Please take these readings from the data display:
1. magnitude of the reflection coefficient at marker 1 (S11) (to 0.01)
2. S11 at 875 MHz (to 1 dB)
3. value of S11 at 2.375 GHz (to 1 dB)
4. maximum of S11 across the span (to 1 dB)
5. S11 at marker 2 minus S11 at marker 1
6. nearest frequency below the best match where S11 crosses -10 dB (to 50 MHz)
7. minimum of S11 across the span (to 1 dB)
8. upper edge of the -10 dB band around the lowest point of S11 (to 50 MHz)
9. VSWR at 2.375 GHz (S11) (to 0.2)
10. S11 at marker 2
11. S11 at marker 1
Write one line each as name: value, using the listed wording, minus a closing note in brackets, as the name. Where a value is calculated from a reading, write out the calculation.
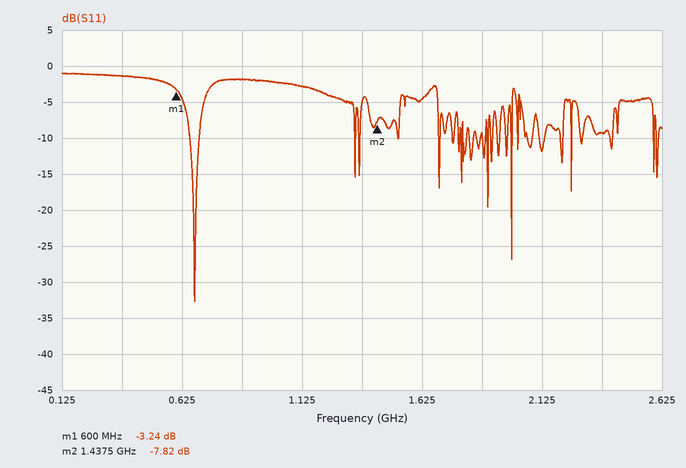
magnitude of the reflection coefficient at marker 1 (S11): 10^(-3.24/20) ≈ 0.69
S11 at 875 MHz: -2 dB
value of S11 at 2.375 GHz: -9 dB
maximum of S11 across the span: -1 dB
S11 at marker 2 minus S11 at marker 1: -7.82 − (-3.24) = -4.58 dB
nearest frequency below the best match where S11 crosses -10 dB: 650 MHz
minimum of S11 across the span: -33 dB
upper edge of the -10 dB band around the lowest point of S11: 700 MHz
VSWR at 2.375 GHz (S11): |Γ| = 10^(-9/20) = 0.3548; VSWR = (1 + 0.3548)/(1 − 0.3548) ≈ 2.10, so 2.0 to the nearest 0.2
S11 at marker 2: -7.82 dB
S11 at marker 1: -3.24 dB
